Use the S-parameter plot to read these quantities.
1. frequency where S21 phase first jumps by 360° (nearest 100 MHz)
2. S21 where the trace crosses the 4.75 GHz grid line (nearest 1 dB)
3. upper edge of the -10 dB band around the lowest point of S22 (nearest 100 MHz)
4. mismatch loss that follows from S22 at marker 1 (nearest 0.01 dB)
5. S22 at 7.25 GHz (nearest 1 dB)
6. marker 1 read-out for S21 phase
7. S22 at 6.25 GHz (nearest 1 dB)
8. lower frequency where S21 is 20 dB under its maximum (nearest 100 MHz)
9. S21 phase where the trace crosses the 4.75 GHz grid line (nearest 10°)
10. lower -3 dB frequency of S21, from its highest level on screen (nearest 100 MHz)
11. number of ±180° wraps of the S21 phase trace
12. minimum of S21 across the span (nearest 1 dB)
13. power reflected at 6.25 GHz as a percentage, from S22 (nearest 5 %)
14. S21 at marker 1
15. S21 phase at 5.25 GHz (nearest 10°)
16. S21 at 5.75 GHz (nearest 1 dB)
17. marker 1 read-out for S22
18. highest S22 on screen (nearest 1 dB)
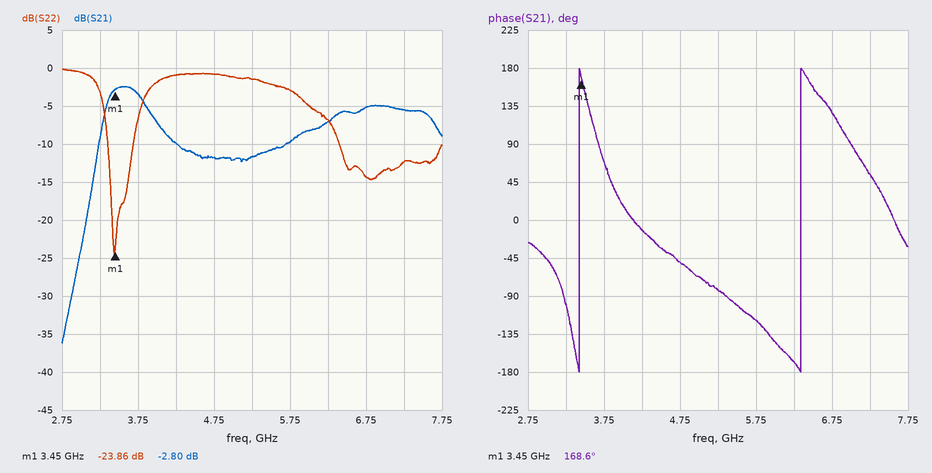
3.4 GHz
-12 dB
3.7 GHz
0.02 dB
-12 dB
168.6°
-7 dB
3.0 GHz
-50°
3.3 GHz
2
-36 dB
20 %
-2.80 dB
-80°
-10 dB
-23.86 dB
0 dB
